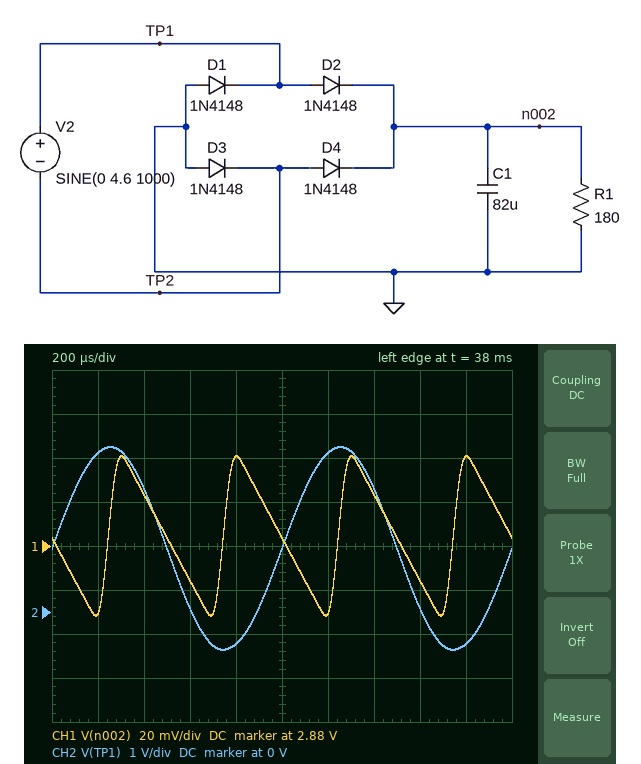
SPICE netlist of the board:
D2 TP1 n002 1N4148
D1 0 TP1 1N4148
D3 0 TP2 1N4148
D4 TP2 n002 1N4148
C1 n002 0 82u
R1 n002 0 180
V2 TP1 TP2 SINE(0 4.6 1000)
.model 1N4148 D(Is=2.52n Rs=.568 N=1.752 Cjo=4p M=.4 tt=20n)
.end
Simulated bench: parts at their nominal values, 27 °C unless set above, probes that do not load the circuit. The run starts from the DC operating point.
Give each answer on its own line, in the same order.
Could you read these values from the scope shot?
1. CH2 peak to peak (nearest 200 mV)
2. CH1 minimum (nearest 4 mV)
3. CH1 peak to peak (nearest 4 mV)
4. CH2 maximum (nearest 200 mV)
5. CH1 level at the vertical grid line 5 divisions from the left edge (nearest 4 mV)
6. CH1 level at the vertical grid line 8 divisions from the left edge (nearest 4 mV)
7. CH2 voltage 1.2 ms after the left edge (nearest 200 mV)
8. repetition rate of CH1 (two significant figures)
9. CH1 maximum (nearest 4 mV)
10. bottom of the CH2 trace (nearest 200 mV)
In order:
4.6 V
2.848 V
72 mV
3.8 V
2.884 V
2.864 V
3.6 V
2.0 kHz
2.920 V
-800 mV
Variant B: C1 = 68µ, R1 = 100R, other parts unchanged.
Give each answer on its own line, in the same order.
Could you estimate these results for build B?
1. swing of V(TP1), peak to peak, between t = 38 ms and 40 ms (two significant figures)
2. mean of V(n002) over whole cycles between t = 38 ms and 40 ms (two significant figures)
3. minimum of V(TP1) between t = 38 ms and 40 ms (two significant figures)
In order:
4.6 V
2.8 V
-910 mV
